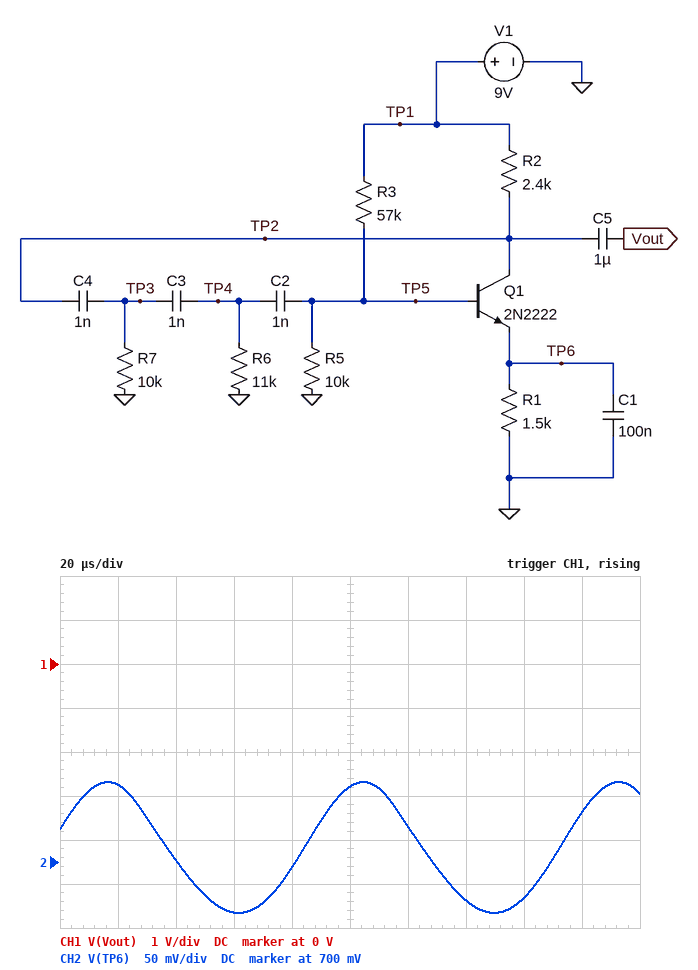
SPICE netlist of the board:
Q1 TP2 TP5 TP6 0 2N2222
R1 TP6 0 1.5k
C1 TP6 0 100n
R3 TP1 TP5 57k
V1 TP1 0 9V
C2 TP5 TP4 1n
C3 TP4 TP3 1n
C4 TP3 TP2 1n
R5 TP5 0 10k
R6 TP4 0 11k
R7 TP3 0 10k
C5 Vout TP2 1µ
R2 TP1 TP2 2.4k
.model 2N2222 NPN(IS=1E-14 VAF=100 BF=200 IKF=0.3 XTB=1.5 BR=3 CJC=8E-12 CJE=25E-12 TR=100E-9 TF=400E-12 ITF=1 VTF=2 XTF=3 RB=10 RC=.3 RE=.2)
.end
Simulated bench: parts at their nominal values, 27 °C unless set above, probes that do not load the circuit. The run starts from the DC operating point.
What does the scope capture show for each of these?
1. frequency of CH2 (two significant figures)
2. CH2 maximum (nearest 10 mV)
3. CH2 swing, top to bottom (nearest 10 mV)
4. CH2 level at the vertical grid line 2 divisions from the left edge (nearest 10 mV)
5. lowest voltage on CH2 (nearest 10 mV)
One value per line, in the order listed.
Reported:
11 kHz
790 mV
150 mV
700 mV
640 mV
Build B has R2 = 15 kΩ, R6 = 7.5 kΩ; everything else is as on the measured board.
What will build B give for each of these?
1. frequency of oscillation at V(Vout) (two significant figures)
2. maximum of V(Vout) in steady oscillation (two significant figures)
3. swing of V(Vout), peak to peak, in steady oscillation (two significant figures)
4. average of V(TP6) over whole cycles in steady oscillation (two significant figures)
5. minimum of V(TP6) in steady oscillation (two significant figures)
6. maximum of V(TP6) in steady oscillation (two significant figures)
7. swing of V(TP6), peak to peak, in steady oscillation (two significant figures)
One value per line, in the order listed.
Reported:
8.0 kHz
4.1 V
3.4 V
670 mV
640 mV
700 mV
63 mV
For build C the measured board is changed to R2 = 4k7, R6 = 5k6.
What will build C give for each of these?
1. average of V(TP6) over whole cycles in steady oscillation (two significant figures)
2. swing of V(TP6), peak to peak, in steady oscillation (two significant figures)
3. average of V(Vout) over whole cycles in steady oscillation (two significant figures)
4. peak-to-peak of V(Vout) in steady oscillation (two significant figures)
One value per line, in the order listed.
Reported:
730 mV
180 mV
6.7 V
4.8 V
